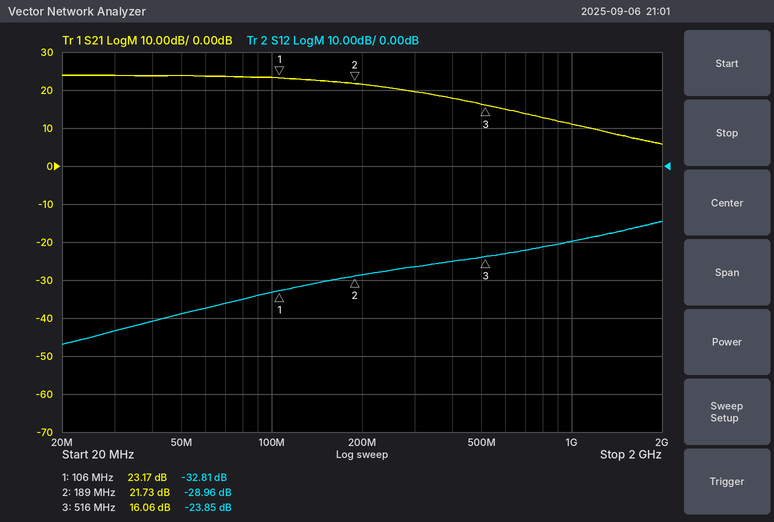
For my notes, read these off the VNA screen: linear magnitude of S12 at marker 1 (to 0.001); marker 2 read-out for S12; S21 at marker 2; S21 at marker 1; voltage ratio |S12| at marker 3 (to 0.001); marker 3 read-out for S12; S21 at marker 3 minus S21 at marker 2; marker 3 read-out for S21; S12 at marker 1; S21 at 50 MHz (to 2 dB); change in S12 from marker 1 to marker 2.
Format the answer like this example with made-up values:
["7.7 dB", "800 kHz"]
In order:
["0.023", "-28.96 dB", "21.73 dB", "23.17 dB", "0.064", "-23.85 dB", "-5.67 dB", "16.06 dB", "-32.81 dB", "24 dB", "3.85 dB"]
